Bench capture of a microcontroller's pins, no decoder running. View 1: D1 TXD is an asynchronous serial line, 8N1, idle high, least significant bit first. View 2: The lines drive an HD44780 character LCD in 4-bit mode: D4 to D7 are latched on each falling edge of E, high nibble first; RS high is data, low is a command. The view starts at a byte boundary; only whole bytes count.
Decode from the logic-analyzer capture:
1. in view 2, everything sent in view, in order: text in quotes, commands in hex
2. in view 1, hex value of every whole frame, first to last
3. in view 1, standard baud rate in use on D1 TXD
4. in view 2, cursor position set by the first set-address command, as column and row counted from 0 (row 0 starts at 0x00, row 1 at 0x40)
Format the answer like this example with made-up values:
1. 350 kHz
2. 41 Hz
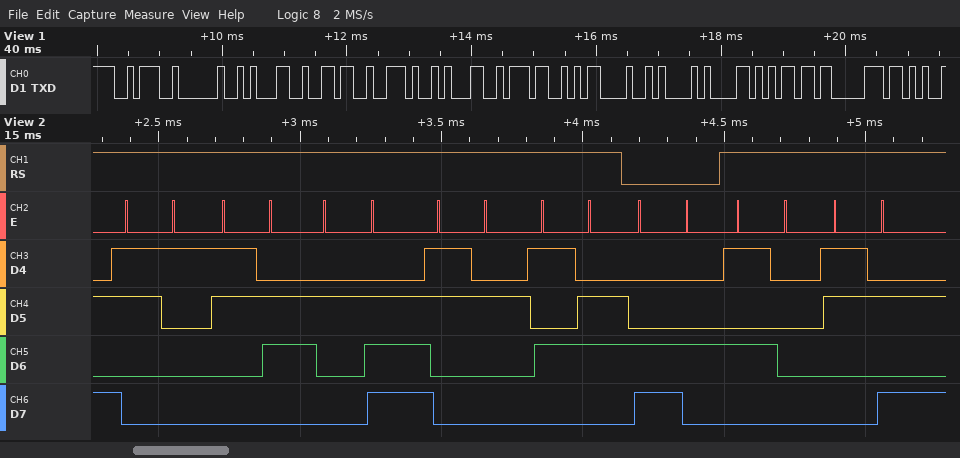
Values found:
1. "16.2V" 0xC4 "P:"
2. 3A 20 31 36 2E 31 37 0D 0A 61 6D 70
3. 9600 baud
4. column 4, row 1
